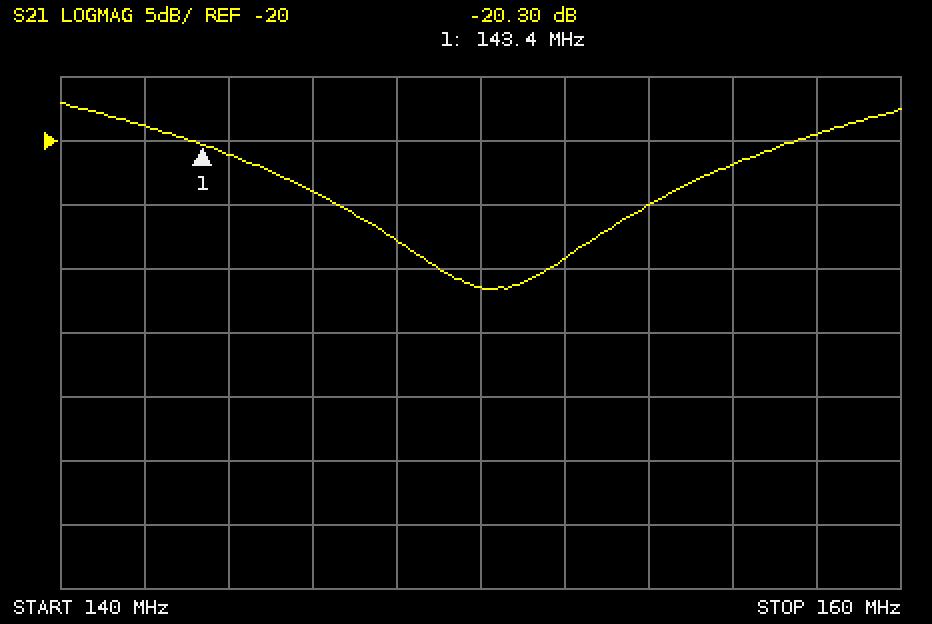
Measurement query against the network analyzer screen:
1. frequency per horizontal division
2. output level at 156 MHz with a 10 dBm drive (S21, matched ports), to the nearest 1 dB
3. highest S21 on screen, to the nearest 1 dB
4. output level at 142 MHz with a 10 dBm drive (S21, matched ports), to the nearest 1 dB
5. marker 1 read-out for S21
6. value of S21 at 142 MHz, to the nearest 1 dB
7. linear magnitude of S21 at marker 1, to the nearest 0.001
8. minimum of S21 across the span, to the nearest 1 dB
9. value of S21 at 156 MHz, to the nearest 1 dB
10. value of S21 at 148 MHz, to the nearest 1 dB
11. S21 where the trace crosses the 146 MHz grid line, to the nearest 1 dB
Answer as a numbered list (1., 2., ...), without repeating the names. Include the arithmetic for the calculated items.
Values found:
1. 2 MHz
2. 10 dBm + (-22 dB) = -12 dBm
3. -17 dB
4. 10 dBm + (-19 dB) = -9 dBm
5. -20.30 dB
6. -19 dB
7. 10^(-20.3/20) ≈ 0.097
8. -32 dB
9. -22 dB
10. -28 dB
11. -24 dB
